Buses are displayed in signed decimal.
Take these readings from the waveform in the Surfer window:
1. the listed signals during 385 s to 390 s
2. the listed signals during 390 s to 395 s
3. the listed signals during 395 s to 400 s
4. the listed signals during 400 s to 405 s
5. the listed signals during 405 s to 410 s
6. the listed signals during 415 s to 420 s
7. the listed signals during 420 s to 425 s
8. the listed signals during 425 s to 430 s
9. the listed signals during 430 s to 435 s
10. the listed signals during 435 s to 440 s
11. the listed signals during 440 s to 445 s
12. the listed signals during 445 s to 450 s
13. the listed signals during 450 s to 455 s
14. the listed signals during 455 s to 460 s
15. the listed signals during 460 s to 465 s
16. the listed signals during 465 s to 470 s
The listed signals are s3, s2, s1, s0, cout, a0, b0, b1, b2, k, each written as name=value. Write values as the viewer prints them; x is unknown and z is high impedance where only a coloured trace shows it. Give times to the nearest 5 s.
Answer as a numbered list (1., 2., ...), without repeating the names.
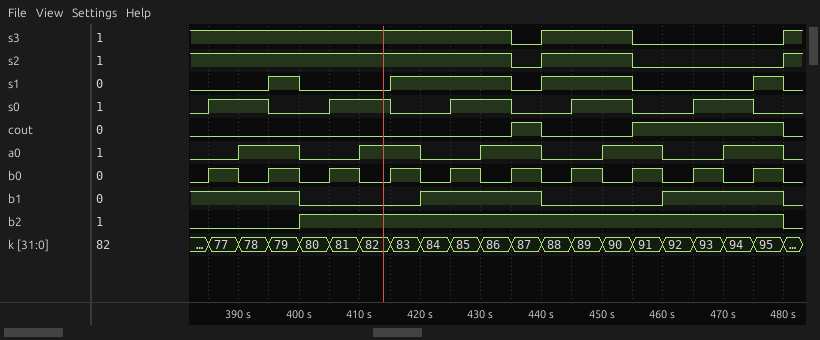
1. s3=1, s2=1, s1=0, s0=1, cout=0, a0=0, b0=1, b1=1, b2=0, k=77
2. s3=1, s2=1, s1=0, s0=1, cout=0, a0=1, b0=0, b1=1, b2=0, k=78
3. s3=1, s2=1, s1=1, s0=0, cout=0, a0=1, b0=1, b1=1, b2=0, k=79
4. s3=1, s2=1, s1=0, s0=0, cout=0, a0=0, b0=0, b1=0, b2=1, k=80
5. s3=1, s2=1, s1=0, s0=1, cout=0, a0=0, b0=1, b1=0, b2=1, k=81
6. s3=1, s2=1, s1=1, s0=0, cout=0, a0=1, b0=1, b1=0, b2=1, k=83
7. s3=1, s2=1, s1=1, s0=0, cout=0, a0=0, b0=0, b1=1, b2=1, k=84
8. s3=1, s2=1, s1=1, s0=1, cout=0, a0=0, b0=1, b1=1, b2=1, k=85
9. s3=1, s2=1, s1=1, s0=1, cout=0, a0=1, b0=0, b1=1, b2=1, k=86
10. s3=0, s2=0, s1=0, s0=0, cout=1, a0=1, b0=1, b1=1, b2=1, k=87
11. s3=1, s2=1, s1=1, s0=0, cout=0, a0=0, b0=0, b1=0, b2=1, k=88
12. s3=1, s2=1, s1=1, s0=1, cout=0, a0=0, b0=1, b1=0, b2=1, k=89
13. s3=1, s2=1, s1=1, s0=1, cout=0, a0=1, b0=0, b1=0, b2=1, k=90
14. s3=0, s2=0, s1=0, s0=0, cout=1, a0=1, b0=1, b1=0, b2=1, k=91
15. s3=0, s2=0, s1=0, s0=0, cout=1, a0=0, b0=0, b1=1, b2=1, k=92
16. s3=0, s2=0, s1=0, s0=1, cout=1, a0=0, b0=1, b1=1, b2=1, k=93
